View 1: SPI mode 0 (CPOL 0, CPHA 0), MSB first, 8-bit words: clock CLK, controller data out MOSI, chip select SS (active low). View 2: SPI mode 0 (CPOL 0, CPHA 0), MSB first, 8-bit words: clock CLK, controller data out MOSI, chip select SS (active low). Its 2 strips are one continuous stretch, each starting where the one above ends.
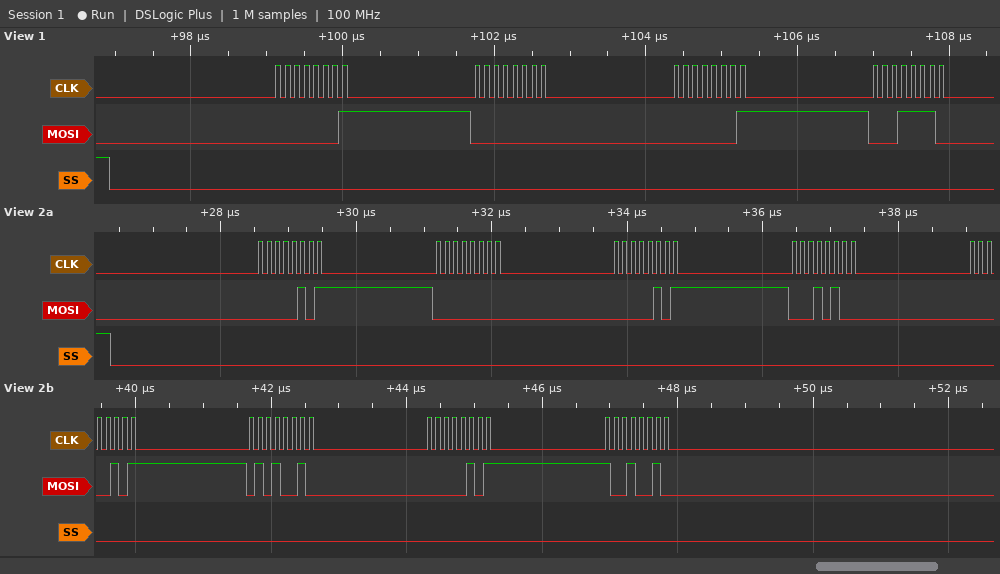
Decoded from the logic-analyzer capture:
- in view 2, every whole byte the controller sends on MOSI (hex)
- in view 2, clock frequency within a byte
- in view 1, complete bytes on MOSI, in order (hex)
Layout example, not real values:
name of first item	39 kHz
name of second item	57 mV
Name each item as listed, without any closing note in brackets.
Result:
in view 2, every whole byte the controller sends on MOSI	05 00 05 14 05 52 05 92
in view 2, clock frequency within a byte	8 MHz
in view 1, complete bytes on MOSI, in order	01 00 01 1E
